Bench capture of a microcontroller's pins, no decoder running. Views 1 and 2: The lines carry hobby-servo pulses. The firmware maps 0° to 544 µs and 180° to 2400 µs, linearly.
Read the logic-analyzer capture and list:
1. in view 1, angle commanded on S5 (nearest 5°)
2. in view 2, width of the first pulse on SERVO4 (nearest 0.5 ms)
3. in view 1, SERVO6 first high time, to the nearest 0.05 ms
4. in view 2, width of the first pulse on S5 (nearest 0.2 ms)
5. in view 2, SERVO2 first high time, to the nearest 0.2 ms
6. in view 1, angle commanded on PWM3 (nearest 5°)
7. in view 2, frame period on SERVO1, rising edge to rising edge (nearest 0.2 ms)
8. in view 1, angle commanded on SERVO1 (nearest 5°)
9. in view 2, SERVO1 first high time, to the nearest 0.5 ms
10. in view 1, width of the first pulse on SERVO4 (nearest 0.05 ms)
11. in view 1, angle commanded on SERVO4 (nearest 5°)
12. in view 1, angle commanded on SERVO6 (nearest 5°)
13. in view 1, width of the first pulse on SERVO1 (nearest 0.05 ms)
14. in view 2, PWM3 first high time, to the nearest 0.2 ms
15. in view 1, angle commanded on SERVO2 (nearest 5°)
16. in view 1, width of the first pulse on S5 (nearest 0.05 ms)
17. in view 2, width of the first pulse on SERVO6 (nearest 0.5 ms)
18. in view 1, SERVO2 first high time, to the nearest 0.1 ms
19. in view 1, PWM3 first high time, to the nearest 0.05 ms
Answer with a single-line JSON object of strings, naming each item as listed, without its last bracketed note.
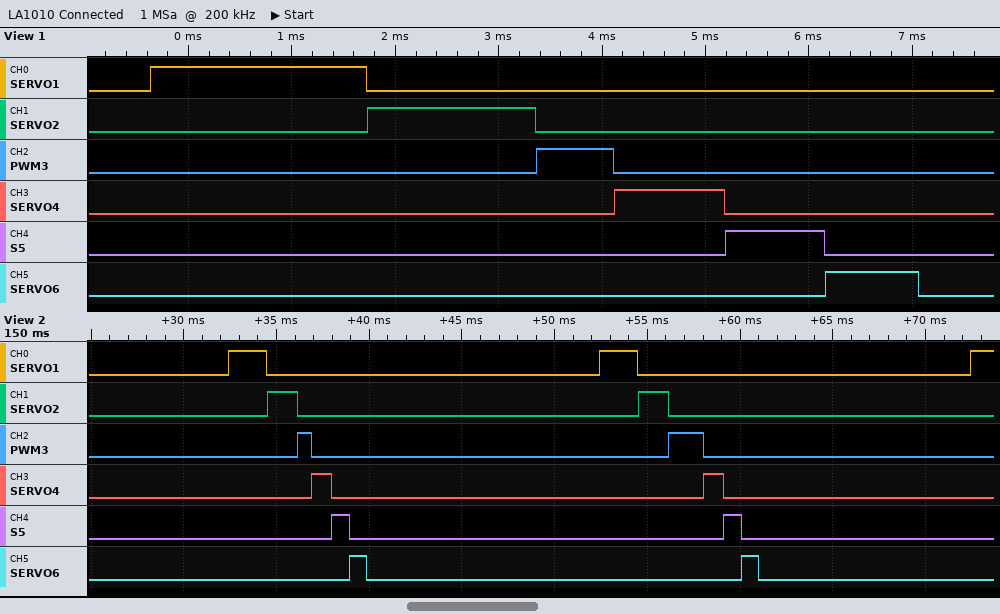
{"in view 1, angle commanded on S5": "40°", "in view 2, width of the first pulse on SERVO4": "1.0 ms", "in view 1, SERVO6 first high time, to the nearest 0.05 ms": "0.90 ms", "in view 2, width of the first pulse on S5": "1.0 ms", "in view 2, SERVO2 first high time, to the nearest 0.2 ms": "1.6 ms", "in view 1, angle commanded on PWM3": "20°", "in view 2, frame period on SERVO1, rising edge to rising edge": "20.0 ms", "in view 1, angle commanded on SERVO1": "150°", "in view 2, SERVO1 first high time, to the nearest 0.5 ms": "2.0 ms", "in view 1, width of the first pulse on SERVO4": "1.05 ms", "in view 1, angle commanded on SERVO4": "50°", "in view 1, angle commanded on SERVO6": "35°", "in view 1, width of the first pulse on SERVO1": "2.10 ms", "in view 2, PWM3 first high time, to the nearest 0.2 ms": "0.8 ms", "in view 1, angle commanded on SERVO2": "105°", "in view 1, width of the first pulse on S5": "0.95 ms", "in view 2, width of the first pulse on SERVO6": "1.0 ms", "in view 1, SERVO2 first high time, to the nearest 0.1 ms": "1.6 ms", "in view 1, PWM3 first high time, to the nearest 0.05 ms": "0.75 ms"}
